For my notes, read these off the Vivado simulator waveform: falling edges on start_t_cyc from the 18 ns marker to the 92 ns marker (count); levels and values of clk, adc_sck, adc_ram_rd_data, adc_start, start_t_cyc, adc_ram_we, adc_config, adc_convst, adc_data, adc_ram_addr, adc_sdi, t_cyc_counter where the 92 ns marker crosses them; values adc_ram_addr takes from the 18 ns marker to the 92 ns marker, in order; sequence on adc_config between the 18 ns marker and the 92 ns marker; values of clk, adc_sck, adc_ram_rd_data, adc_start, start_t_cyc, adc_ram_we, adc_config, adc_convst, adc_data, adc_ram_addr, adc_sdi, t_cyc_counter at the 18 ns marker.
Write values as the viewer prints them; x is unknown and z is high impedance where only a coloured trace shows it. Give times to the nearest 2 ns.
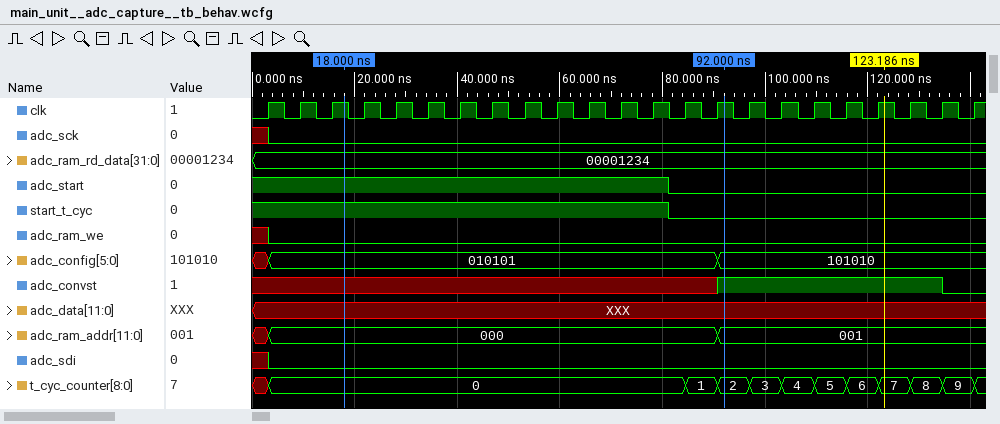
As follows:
1
clk=1, adc_sck=0, adc_ram_rd_data=00001234, adc_start=0, start_t_cyc=0, adc_ram_we=0, adc_config=101010, adc_convst=1, adc_data=XXX, adc_ram_addr=001, adc_sdi=0, t_cyc_counter=2
000, 001
010101, 101010
clk=1, adc_sck=0, adc_ram_rd_data=00001234, adc_start=1, start_t_cyc=1, adc_ram_we=0, adc_config=010101, adc_convst=x, adc_data=XXX, adc_ram_addr=000, adc_sdi=0, t_cyc_counter=0
